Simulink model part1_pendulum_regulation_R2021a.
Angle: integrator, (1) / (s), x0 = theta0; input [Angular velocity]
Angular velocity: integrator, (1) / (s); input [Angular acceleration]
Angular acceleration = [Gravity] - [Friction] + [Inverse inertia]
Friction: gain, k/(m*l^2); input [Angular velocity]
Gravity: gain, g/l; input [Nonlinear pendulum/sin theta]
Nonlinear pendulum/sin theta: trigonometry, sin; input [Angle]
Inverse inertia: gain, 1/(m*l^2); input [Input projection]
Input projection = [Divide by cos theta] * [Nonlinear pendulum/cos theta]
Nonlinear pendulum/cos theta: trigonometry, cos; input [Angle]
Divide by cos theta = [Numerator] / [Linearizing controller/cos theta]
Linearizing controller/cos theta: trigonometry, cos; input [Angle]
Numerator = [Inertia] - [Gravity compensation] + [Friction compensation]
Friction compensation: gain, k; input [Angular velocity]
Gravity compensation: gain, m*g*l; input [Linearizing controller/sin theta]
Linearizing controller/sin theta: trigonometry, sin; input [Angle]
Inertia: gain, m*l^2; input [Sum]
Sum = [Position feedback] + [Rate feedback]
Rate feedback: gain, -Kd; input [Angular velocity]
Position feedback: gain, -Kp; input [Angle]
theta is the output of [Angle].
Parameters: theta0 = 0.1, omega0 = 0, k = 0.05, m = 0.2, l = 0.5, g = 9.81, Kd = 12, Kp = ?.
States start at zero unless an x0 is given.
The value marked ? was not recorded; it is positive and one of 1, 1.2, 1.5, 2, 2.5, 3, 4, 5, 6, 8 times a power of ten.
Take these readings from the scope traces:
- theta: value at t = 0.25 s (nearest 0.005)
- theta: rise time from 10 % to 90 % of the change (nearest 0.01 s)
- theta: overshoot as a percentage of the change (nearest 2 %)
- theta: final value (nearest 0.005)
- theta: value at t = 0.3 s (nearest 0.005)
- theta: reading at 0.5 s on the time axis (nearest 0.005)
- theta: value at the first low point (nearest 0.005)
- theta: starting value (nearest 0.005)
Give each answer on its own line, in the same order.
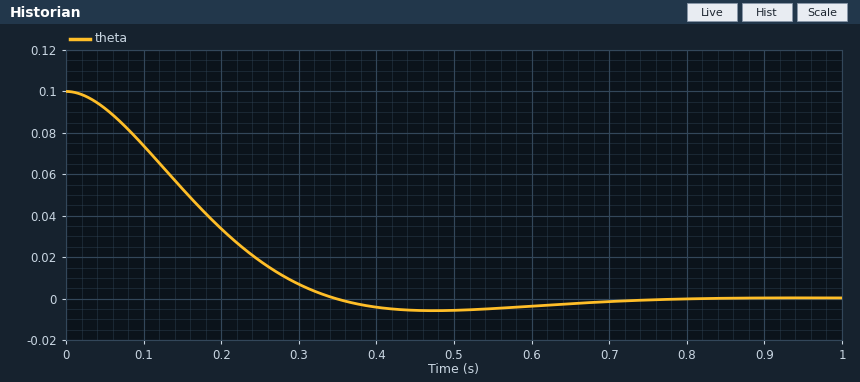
0.020
0.23 s
6 %
0.000
0.005
-0.005
-0.005
0.100
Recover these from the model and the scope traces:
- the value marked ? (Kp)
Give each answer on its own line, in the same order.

80
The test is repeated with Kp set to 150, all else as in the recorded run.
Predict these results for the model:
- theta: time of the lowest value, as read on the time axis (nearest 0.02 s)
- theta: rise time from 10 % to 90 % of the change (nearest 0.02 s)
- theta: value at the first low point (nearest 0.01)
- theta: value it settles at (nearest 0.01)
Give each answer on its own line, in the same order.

0.30 s
0.14 s
-0.02
0.00
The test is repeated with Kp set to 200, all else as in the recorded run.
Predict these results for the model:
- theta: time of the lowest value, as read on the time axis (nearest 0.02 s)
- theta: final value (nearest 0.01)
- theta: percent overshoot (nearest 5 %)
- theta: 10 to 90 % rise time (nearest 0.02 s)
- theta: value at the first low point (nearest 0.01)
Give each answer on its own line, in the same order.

0.24 s
0.00
25 %
0.10 s
-0.02
